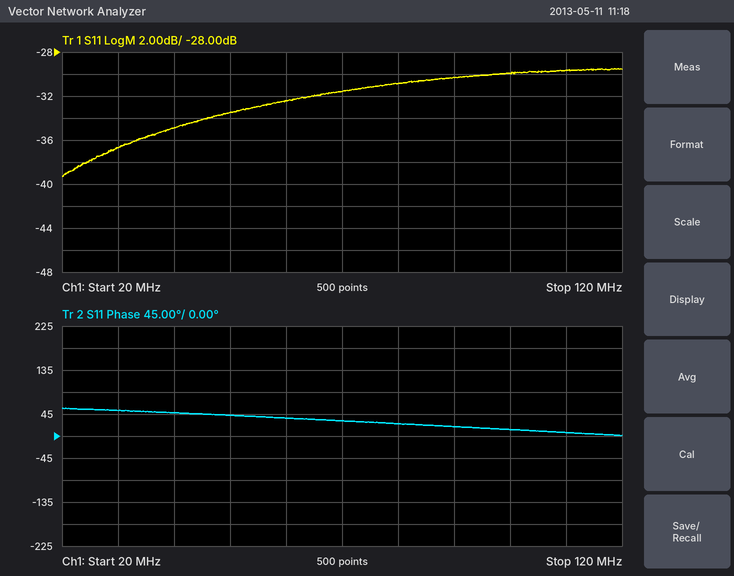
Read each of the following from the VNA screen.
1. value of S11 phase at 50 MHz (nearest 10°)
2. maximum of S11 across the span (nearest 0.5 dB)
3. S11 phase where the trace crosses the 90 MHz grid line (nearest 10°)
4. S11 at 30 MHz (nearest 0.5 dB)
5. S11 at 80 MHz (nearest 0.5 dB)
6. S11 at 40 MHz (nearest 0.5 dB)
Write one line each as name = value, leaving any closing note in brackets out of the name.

value of S11 phase at 50 MHz = 40°
maximum of S11 across the span = -29.5 dB
S11 phase where the trace crosses the 90 MHz grid line = 20°
S11 at 30 MHz = -36.5 dB
S11 at 80 MHz = -31.0 dB
S11 at 40 MHz = -35.0 dB
